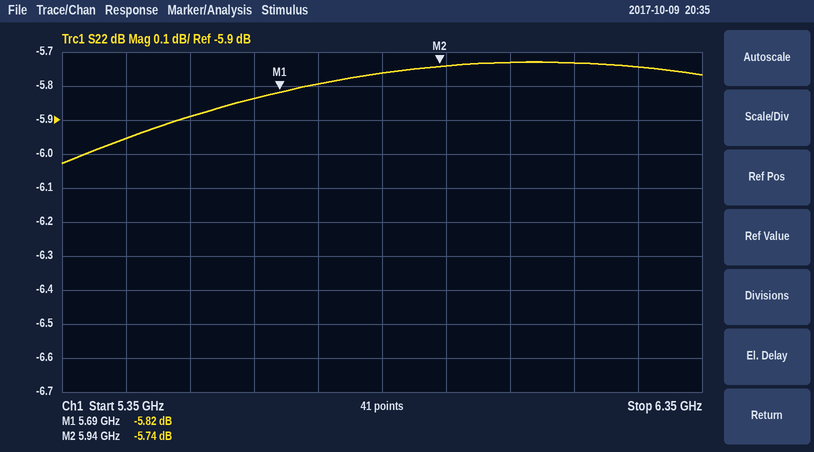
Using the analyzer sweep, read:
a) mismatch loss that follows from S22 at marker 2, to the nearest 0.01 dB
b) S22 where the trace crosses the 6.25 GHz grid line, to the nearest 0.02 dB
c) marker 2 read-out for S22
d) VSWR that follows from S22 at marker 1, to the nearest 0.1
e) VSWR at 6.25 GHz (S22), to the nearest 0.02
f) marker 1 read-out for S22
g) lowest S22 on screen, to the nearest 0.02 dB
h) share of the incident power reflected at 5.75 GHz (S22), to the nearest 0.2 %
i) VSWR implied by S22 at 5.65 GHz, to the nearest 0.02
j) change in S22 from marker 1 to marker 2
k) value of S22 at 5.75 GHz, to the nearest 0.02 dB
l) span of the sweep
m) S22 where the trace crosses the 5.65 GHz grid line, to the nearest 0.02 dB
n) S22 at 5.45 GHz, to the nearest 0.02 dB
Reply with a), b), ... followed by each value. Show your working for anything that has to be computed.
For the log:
a) −10 log10(1 − 10^(-5.74/10)) ≈ 1.35 dB
b) -5.74 dB
c) -5.74 dB
d) (1 + 0.5117)/(1 − 0.5117) ≈ 3.1
e) |Γ| = 10^(-5.74/20) = 0.5164; VSWR = (1 + 0.5164)/(1 − 0.5164) ≈ 3.14
f) -5.82 dB
g) -6.02 dB
h) 10^(-5.8/10) ≈ 26.3 %, so 26.4 % to the nearest 0.2 %
i) |Γ| = 10^(-5.84/20) = 0.5105; VSWR = (1 + 0.5105)/(1 − 0.5105) ≈ 3.09, so 3.08 to the nearest 0.02
j) -5.74 − (-5.82) = 0.08 dB
k) -5.80 dB
l) 1 GHz
m) -5.84 dB
n) -5.96 dB
